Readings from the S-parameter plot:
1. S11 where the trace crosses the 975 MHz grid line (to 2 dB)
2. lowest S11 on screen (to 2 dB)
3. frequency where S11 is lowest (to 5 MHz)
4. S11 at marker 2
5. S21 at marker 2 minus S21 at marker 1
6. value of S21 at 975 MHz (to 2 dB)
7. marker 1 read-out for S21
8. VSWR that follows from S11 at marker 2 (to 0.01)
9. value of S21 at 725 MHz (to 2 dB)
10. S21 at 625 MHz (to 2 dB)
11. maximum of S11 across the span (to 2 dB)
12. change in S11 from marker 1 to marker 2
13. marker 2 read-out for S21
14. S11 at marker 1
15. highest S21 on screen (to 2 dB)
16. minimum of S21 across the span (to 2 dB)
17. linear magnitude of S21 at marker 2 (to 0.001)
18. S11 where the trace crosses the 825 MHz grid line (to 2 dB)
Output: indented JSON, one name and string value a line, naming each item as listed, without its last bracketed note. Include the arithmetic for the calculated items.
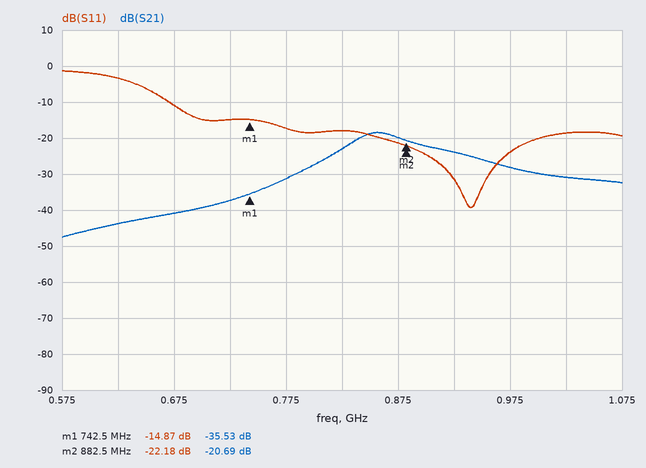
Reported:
{
  "S11 where the trace crosses the 975 MHz grid line": "-24 dB",
  "lowest S11 on screen": "-40 dB",
  "frequency where S11 is lowest": "940 MHz",
  "S11 at marker 2": "-22.18 dB",
  "S21 at marker 2 minus S21 at marker 1": "-20.69 − (-35.53) = 14.84 dB",
  "value of S21 at 975 MHz": "-28 dB",
  "marker 1 read-out for S21": "-35.53 dB",
  "VSWR that follows from S11 at marker 2": "(1 + 0.0778)/(1 − 0.0778) ≈ 1.17",
  "value of S21 at 725 MHz": "-38 dB",
  "S21 at 625 MHz": "-44 dB",
  "maximum of S11 across the span": "-2 dB",
  "change in S11 from marker 1 to marker 2": "-22.18 − (-14.87) = -7.31 dB",
  "marker 2 read-out for S21": "-20.69 dB",
  "S11 at marker 1": "-14.87 dB",
  "highest S21 on screen": "-18 dB",
  "minimum of S21 across the span": "-48 dB",
  "linear magnitude of S21 at marker 2": "10^(-20.69/20) ≈ 0.092",
  "S11 where the trace crosses the 825 MHz grid line": "-18 dB"
}
